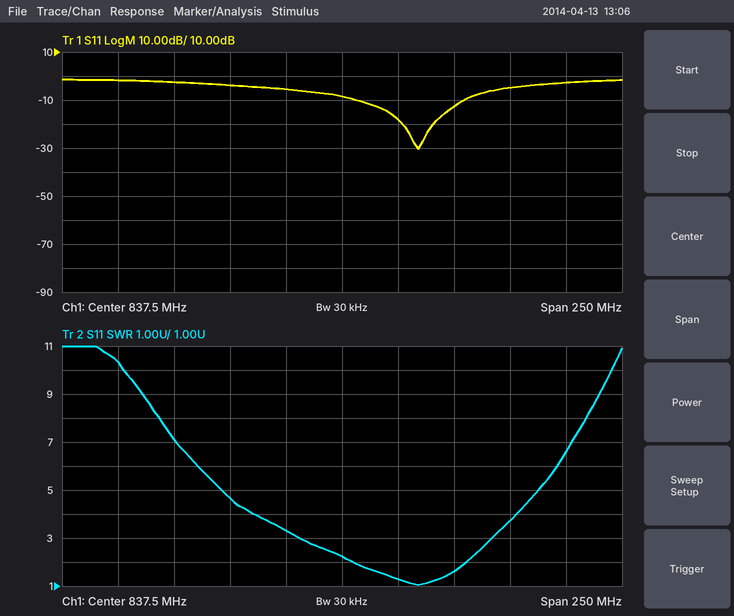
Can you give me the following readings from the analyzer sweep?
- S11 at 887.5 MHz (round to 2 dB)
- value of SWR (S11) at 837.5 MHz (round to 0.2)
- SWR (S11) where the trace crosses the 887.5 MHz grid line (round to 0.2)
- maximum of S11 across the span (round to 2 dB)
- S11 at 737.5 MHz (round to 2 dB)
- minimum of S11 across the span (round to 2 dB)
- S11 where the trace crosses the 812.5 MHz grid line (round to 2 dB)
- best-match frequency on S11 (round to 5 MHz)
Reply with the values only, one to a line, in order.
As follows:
-12 dB
2.2
1.6
-2 dB
-2 dB
-30 dB
-6 dB
870 MHz
